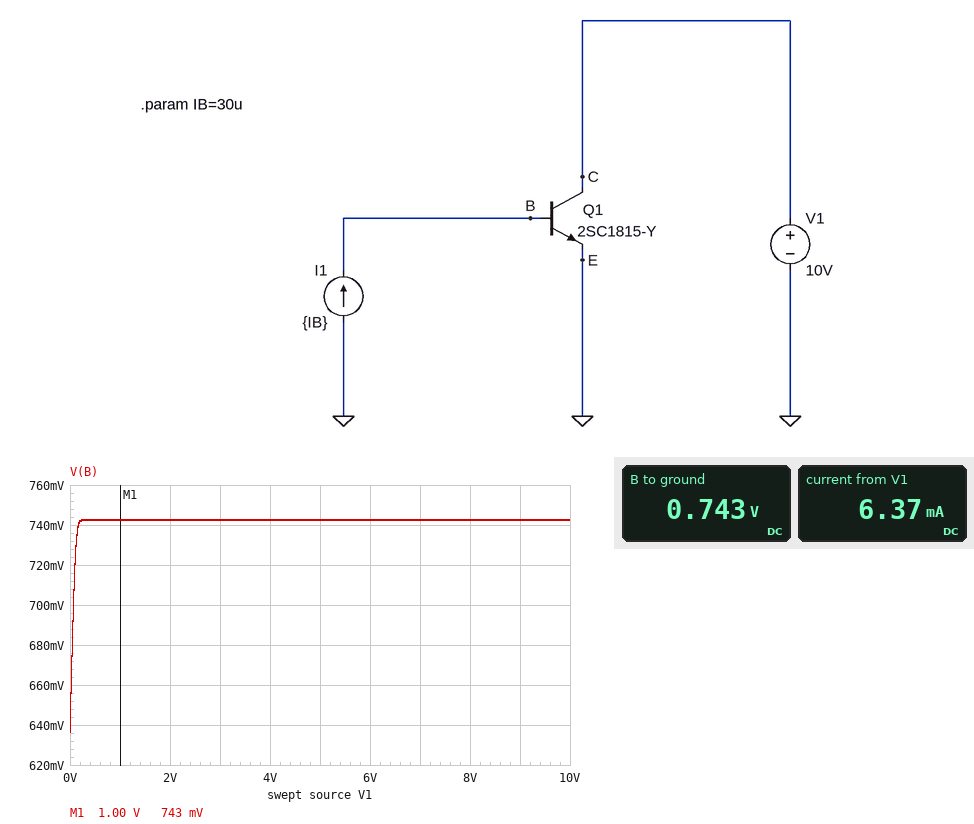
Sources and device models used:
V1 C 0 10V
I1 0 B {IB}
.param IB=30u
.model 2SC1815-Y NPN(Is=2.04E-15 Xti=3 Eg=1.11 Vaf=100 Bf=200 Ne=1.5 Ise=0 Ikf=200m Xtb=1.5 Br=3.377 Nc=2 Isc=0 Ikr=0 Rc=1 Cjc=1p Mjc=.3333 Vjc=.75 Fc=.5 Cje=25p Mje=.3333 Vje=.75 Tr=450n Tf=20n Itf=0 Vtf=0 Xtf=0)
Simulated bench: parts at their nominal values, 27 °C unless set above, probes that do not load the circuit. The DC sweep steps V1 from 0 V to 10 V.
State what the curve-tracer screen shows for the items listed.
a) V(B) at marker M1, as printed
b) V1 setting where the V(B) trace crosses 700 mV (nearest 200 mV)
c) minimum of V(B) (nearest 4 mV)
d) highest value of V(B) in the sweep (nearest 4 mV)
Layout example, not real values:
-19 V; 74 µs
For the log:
743 mV; 0 V; 636 mV; 744 mV
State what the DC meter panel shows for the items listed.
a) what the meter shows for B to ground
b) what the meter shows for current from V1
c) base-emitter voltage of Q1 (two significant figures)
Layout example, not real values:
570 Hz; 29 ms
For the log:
0.743 V; 6.37 mA; 740 mV
